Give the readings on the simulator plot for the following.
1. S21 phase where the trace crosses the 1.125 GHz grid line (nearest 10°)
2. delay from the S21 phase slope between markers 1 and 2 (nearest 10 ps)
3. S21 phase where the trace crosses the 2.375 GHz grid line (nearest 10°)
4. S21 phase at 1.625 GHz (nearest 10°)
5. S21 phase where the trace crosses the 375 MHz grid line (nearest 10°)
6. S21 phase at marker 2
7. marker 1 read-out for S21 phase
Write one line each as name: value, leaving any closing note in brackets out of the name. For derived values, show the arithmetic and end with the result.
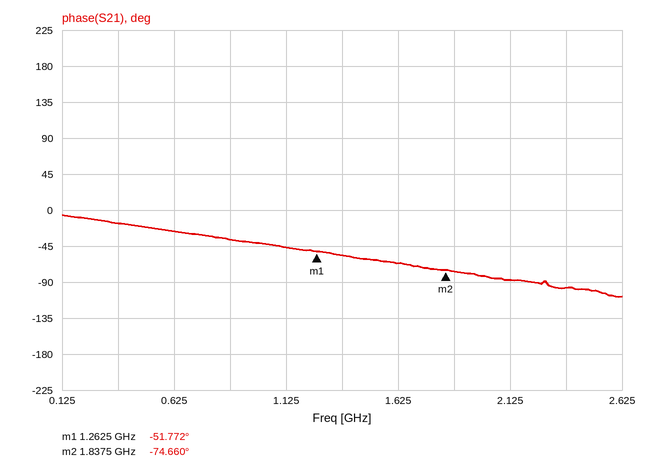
S21 phase where the trace crosses the 1.125 GHz grid line: -50°
delay from the S21 phase slope between markers 1 and 2: −(-74.66° − (-51.772°))/(360° × 575 MHz) ≈ 111 ps, so 110 ps to the nearest 10 ps
S21 phase where the trace crosses the 2.375 GHz grid line: -100°
S21 phase at 1.625 GHz: -70°
S21 phase where the trace crosses the 375 MHz grid line: -20°
S21 phase at marker 2: -74.660°
marker 1 read-out for S21 phase: -51.772°
